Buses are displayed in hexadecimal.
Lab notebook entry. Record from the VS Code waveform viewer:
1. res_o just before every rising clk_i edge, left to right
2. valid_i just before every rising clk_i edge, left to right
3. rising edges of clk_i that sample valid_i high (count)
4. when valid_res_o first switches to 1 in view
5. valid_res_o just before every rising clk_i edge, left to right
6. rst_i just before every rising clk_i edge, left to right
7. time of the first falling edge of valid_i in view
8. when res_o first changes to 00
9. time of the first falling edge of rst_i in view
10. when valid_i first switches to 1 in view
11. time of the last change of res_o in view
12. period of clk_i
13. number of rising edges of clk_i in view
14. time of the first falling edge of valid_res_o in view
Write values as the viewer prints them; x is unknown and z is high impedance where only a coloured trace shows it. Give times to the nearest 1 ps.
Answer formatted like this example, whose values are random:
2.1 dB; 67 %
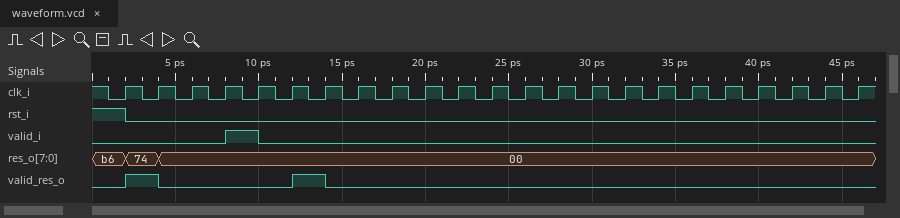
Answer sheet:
b6, 74, 00, 00, 00, 00, 00, 00, 00, 00, 00, 00, 00, 00, 00, 00, 00, 00, 00, 00, 00, 00, 00; 0 0 0 0 1 0 0 0 0 0 0 0 0 0 0 0 0 0 0 0 0 0 0; 1; 2 ps; 0 1 0 0 0 0 1 0 0 0 0 0 0 0 0 0 0 0 0 0 0 0 0; 1 0 0 0 0 0 0 0 0 0 0 0 0 0 0 0 0 0 0 0 0 0 0; 10 ps; 4 ps; 2 ps; 8 ps; 4 ps; 2 ps; 23; 4 ps
